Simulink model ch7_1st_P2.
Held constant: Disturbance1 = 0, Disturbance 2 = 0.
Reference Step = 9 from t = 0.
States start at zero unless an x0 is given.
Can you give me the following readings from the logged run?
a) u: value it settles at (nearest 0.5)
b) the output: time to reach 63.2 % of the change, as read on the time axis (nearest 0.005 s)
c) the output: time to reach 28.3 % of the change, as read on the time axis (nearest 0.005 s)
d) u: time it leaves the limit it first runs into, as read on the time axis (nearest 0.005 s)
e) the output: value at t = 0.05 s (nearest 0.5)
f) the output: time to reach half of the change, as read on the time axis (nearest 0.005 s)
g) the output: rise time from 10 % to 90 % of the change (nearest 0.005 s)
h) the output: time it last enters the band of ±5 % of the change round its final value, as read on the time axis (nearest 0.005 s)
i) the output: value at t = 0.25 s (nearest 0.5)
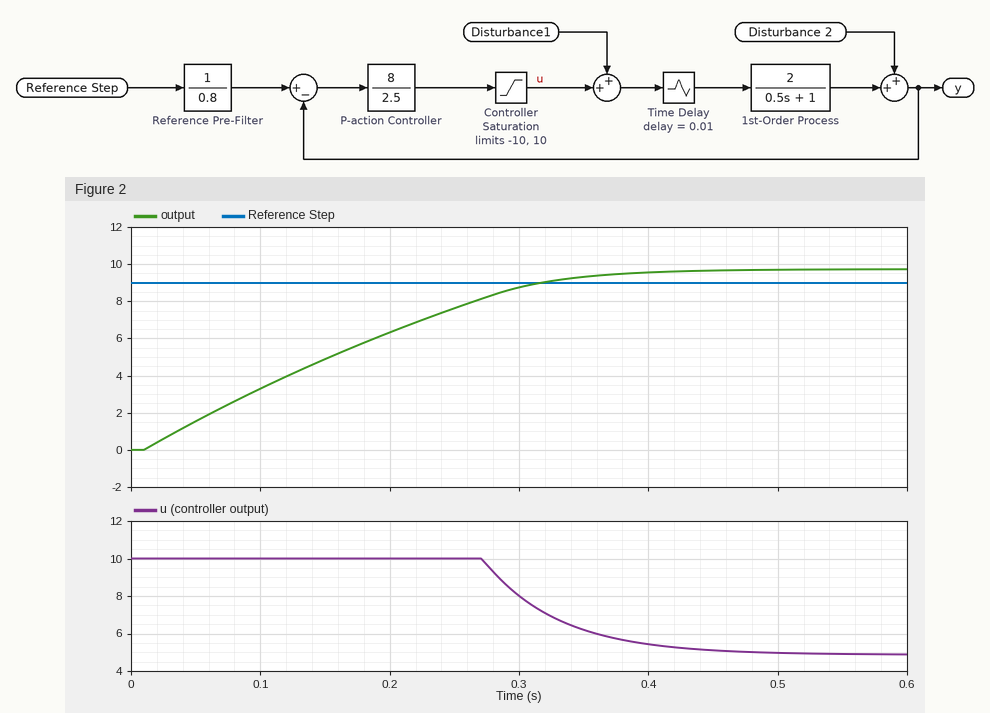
5.0
0.195 s
0.085 s
0.270 s
1.5
0.150 s
0.265 s
0.340 s
7.5
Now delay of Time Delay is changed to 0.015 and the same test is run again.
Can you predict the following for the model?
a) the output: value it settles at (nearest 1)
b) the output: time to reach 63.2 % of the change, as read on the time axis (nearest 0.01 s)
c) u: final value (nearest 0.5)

10
0.20 s
5.0
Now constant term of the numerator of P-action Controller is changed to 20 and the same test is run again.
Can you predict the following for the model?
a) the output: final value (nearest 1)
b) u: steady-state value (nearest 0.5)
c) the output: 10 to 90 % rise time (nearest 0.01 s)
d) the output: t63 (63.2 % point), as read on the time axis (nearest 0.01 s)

11
5.5
0.30 s
0.21 s
